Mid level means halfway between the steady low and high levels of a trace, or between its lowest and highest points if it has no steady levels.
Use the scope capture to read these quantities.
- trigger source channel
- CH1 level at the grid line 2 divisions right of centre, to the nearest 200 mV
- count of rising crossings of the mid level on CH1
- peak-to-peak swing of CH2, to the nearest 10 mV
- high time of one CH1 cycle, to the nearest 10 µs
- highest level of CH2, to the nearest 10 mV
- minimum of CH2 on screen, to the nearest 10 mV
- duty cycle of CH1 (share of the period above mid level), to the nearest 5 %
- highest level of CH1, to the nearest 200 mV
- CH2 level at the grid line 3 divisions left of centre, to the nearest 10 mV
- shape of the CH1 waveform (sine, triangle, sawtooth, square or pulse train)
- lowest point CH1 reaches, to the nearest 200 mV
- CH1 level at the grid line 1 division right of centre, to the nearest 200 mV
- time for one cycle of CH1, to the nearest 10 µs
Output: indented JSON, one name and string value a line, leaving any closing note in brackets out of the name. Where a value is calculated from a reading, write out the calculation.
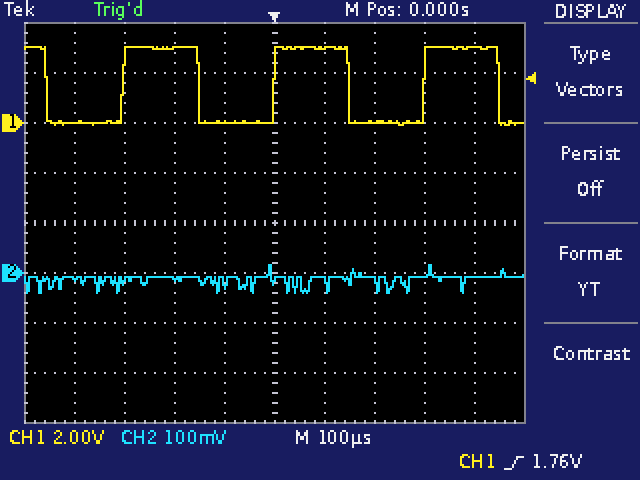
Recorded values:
{
  "trigger source channel": "CH1",
  "CH1 level at the grid line 2 divisions right of centre, to the nearest 200 mV": "0.0 V",
  "count of rising crossings of the mid level on CH1": "3",
  "peak-to-peak swing of CH2, to the nearest 10 mV": "20 mV − (-40 mV) = 60 mV",
  "high time of one CH1 cycle, to the nearest 10 µs": "150 µs",
  "highest level of CH2, to the nearest 10 mV": "20 mV",
  "minimum of CH2 on screen, to the nearest 10 mV": "-40 mV",
  "duty cycle of CH1 (share of the period above mid level), to the nearest 5 %": "150 µs / 300 µs ≈ 50 %",
  "highest level of CH1, to the nearest 200 mV": "3.0 V",
  "CH2 level at the grid line 3 divisions left of centre, to the nearest 10 mV": "-20 mV",
  "shape of the CH1 waveform": "square",
  "lowest point CH1 reaches, to the nearest 200 mV": "0.0 V",
  "CH1 level at the grid line 1 division right of centre, to the nearest 200 mV": "3.0 V",
  "time for one cycle of CH1, to the nearest 10 µs": "300 µs"
}
